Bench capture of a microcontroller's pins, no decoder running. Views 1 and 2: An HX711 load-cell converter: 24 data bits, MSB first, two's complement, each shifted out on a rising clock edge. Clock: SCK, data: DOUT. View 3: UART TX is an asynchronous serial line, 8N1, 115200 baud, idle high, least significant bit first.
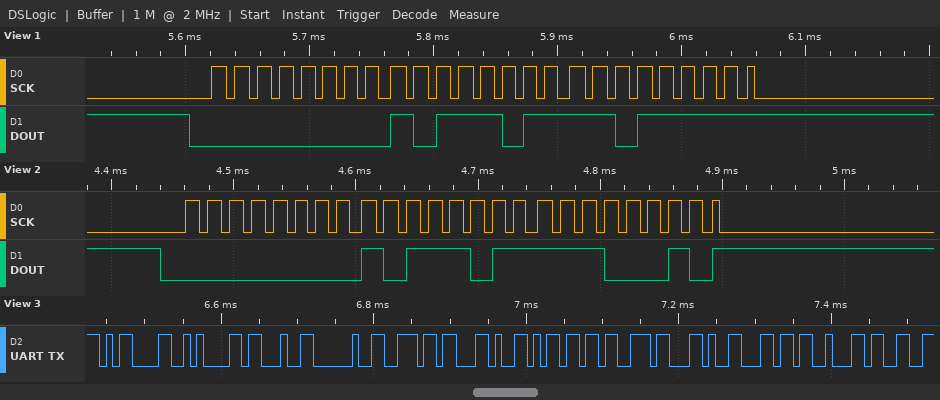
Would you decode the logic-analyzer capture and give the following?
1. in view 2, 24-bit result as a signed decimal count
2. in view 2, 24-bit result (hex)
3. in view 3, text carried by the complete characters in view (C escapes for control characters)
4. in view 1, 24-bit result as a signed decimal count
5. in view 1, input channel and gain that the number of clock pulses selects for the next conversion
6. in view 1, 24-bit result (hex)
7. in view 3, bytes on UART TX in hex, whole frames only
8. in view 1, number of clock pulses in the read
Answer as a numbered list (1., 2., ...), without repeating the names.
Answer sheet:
1. 48098
2. 0x00BBE2
3. "\r\n# n,ms,lb"
4. 48095
5. channel A, gain 128
6. 0x00BBDF
7. 0D 0A 23 20 6E 2C 6D 73 2C 6C 62
8. 25
